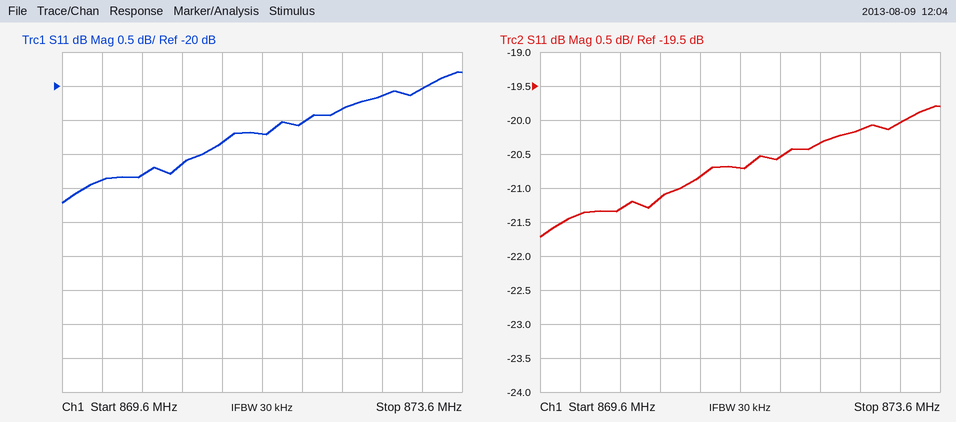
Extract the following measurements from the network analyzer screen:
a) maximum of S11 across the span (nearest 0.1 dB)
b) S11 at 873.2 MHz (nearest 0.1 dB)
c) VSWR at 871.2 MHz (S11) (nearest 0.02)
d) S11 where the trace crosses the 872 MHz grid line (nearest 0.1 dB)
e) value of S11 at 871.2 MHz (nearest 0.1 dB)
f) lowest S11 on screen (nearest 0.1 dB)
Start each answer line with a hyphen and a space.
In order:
- -19.8 dB
- -20.0 dB
- 1.20
- -20.5 dB
- -20.8 dB
- -21.7 dB
